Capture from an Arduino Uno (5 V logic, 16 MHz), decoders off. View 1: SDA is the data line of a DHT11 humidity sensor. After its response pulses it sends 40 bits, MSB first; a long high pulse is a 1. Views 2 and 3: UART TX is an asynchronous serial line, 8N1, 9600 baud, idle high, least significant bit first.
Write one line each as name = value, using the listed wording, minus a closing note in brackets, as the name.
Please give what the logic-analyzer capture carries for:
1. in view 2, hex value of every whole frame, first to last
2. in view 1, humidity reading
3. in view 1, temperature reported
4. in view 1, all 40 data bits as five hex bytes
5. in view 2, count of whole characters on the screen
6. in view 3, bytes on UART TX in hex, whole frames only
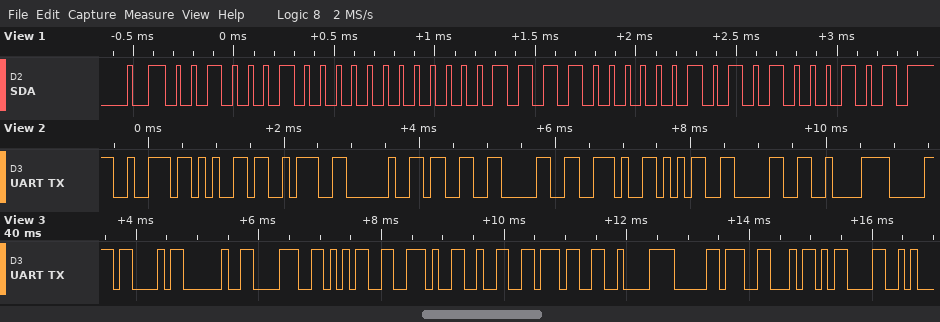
in view 2, hex value of every whole frame, first to last = 72 65 3A 20 33 30 2E 35 30 C2
in view 1, humidity reading = 34 %
in view 1, temperature reported = 30.5 °C
in view 1, all 40 data bits as five hex bytes = 22 00 1E 05 45
in view 2, count of whole characters on the screen = 10
in view 3, bytes on UART TX in hex, whole frames only = 43 20 38 35 2E 32 37 C2 B0 46 0D
